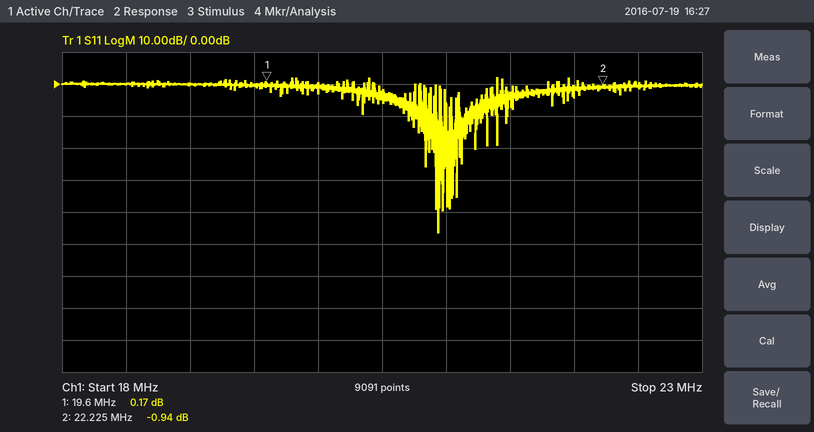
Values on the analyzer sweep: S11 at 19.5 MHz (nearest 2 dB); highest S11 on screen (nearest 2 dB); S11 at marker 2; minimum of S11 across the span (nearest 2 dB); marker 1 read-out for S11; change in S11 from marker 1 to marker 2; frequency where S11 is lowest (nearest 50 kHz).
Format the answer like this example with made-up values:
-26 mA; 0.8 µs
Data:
0 dB; 2 dB; -0.94 dB; -46 dB; 0.17 dB; -1.11 dB; 20.95 MHz
